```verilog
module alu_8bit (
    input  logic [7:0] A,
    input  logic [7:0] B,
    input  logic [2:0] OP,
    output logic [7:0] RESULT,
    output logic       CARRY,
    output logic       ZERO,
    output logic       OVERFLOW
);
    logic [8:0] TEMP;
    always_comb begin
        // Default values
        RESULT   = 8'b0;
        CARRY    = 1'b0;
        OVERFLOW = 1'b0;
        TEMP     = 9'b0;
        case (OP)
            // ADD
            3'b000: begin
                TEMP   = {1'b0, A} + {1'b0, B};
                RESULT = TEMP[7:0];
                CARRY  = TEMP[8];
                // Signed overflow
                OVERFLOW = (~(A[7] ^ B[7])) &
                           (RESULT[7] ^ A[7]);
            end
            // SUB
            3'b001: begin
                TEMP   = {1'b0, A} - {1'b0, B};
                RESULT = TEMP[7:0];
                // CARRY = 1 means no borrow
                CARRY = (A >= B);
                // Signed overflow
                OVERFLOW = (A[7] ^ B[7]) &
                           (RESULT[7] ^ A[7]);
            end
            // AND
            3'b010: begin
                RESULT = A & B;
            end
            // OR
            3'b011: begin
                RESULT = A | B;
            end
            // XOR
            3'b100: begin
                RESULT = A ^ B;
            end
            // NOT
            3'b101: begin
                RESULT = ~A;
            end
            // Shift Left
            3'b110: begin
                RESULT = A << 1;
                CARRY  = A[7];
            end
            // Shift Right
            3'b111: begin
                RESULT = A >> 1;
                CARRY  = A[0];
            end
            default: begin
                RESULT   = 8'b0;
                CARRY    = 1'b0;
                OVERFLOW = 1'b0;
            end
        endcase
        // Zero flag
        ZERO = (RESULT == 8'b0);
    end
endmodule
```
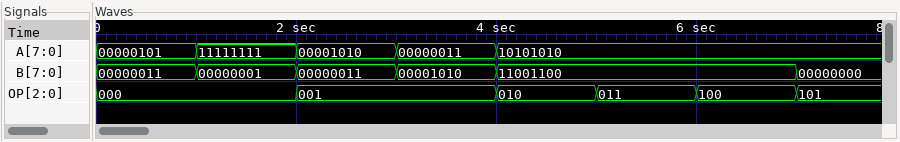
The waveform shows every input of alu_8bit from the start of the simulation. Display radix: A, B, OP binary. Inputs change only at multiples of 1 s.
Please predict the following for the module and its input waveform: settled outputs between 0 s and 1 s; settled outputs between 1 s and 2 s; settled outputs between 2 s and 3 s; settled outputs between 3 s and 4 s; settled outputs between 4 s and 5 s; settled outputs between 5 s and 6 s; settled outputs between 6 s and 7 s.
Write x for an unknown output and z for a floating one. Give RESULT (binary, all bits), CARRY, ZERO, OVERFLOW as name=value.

RESULT=00001000, CARRY=0, ZERO=0, OVERFLOW=0
RESULT=00000000, CARRY=1, ZERO=1, OVERFLOW=0
RESULT=00000111, CARRY=1, ZERO=0, OVERFLOW=0
RESULT=11111001, CARRY=0, ZERO=0, OVERFLOW=0
RESULT=10001000, CARRY=0, ZERO=0, OVERFLOW=0
RESULT=11101110, CARRY=0, ZERO=0, OVERFLOW=0
RESULT=01100110, CARRY=0, ZERO=0, OVERFLOW=0
